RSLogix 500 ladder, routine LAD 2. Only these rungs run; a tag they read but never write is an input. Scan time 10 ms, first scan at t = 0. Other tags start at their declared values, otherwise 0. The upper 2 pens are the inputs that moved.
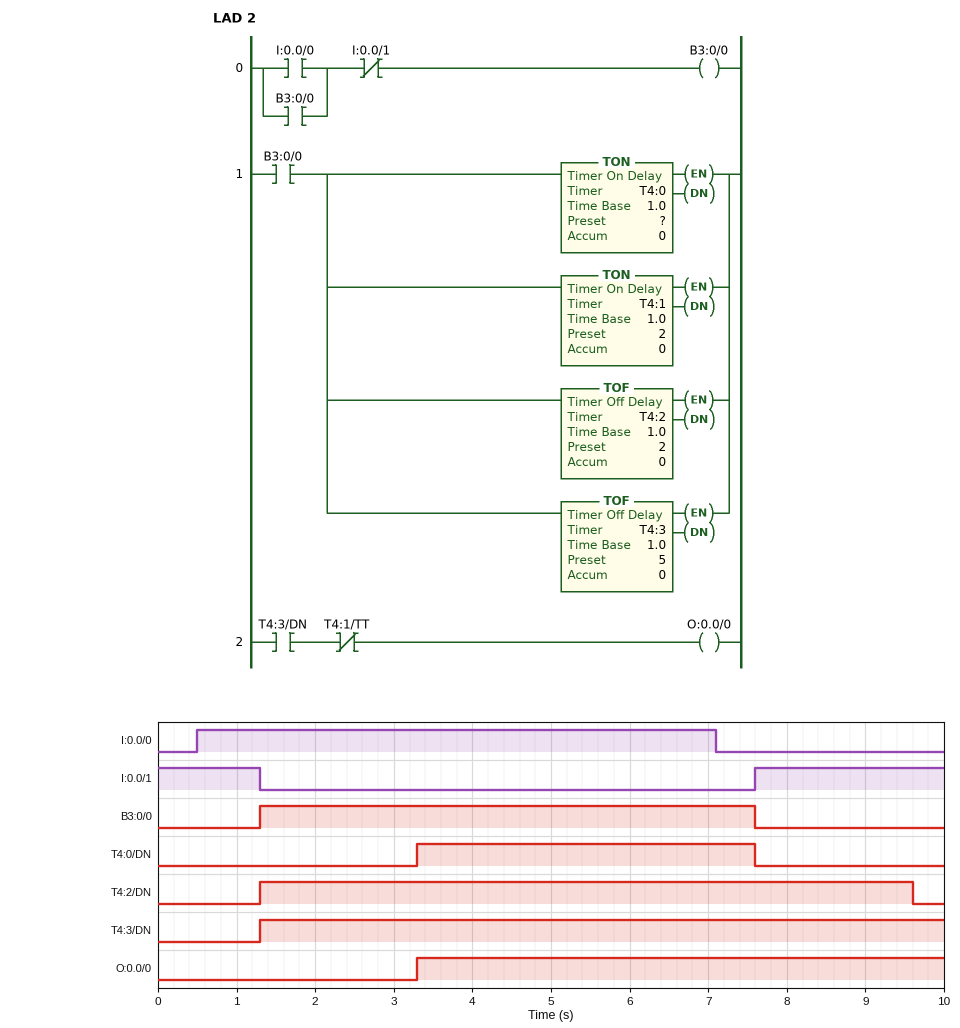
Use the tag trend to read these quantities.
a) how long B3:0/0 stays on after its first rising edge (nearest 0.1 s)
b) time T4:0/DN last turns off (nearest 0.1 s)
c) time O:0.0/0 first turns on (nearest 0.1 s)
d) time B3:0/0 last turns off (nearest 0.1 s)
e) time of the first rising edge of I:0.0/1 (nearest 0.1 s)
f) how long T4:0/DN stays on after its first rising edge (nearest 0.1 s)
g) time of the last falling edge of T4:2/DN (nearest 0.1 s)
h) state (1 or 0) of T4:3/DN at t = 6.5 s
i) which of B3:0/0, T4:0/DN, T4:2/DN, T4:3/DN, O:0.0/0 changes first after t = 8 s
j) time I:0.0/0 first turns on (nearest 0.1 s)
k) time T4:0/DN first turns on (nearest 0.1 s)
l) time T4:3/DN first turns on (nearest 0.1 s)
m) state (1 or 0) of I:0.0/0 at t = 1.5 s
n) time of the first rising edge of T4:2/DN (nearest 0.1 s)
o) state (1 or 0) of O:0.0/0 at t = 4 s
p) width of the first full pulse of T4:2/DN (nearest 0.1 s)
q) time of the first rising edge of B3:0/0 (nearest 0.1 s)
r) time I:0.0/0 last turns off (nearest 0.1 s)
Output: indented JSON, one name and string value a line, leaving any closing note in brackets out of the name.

{
  "how long B3:0/0 stays on after its first rising edge": "6.3 s",
  "time T4:0/DN last turns off": "7.6 s",
  "time O:0.0/0 first turns on": "3.3 s",
  "time B3:0/0 last turns off": "7.6 s",
  "time of the first rising edge of I:0.0/1": "7.6 s",
  "how long T4:0/DN stays on after its first rising edge": "4.3 s",
  "time of the last falling edge of T4:2/DN": "9.6 s",
  "state (1 or 0) of T4:3/DN at t = 6.5 s": "1",
  "which of B3:0/0, T4:0/DN, T4:2/DN, T4:3/DN, O:0.0/0 changes first after t = 8 s": "T4:2/DN",
  "time I:0.0/0 first turns on": "0.5 s",
  "time T4:0/DN first turns on": "3.3 s",
  "time T4:3/DN first turns on": "1.3 s",
  "state (1 or 0) of I:0.0/0 at t = 1.5 s": "1",
  "time of the first rising edge of T4:2/DN": "1.3 s",
  "state (1 or 0) of O:0.0/0 at t = 4 s": "1",
  "width of the first full pulse of T4:2/DN": "8.3 s",
  "time of the first rising edge of B3:0/0": "1.3 s",
  "time I:0.0/0 last turns off": "7.1 s"
}
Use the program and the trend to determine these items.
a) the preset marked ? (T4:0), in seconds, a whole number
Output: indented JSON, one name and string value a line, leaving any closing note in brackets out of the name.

{
  "the preset marked ? (T4:0), in seconds, a whole number": "2 s"
}
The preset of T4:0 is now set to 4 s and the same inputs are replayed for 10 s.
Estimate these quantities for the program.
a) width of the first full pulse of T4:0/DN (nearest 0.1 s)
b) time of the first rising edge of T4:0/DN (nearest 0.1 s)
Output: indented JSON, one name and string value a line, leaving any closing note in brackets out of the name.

{
  "width of the first full pulse of T4:0/DN": "2.3 s",
  "time of the first rising edge of T4:0/DN": "5.3 s"
}
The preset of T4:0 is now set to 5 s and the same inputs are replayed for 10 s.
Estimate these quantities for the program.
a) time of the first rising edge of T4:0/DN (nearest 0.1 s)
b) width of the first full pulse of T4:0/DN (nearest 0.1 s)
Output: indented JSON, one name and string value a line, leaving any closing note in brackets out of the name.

{
  "time of the first rising edge of T4:0/DN": "6.3 s",
  "width of the first full pulse of T4:0/DN": "1.3 s"
}
